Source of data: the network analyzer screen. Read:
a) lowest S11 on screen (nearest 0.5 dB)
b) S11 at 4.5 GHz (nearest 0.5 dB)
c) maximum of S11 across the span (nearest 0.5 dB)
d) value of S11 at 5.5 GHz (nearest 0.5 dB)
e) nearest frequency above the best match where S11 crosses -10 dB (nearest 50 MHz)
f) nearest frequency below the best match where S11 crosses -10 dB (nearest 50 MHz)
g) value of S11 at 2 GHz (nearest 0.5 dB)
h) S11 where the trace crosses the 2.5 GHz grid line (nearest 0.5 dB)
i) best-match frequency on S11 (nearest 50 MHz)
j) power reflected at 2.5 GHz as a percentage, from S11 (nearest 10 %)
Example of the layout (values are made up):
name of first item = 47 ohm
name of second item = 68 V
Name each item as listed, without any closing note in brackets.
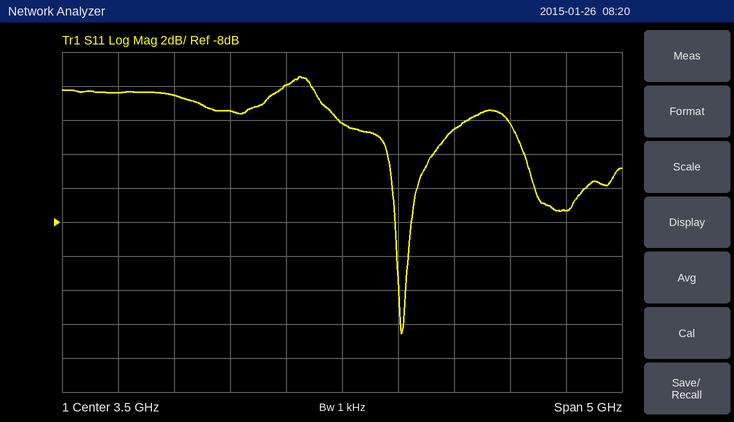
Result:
lowest S11 on screen = -14.5 dB
S11 at 4.5 GHz = -2.5 dB
maximum of S11 across the span = 0.5 dB
value of S11 at 5.5 GHz = -7.5 dB
nearest frequency above the best match where S11 crosses -10 dB = 4.10 GHz
nearest frequency below the best match where S11 crosses -10 dB = 4.00 GHz
value of S11 at 2 GHz = -0.5 dB
S11 where the trace crosses the 2.5 GHz grid line = -1.5 dB
best-match frequency on S11 = 4.05 GHz
power reflected at 2.5 GHz as a percentage, from S11 = 70 %
